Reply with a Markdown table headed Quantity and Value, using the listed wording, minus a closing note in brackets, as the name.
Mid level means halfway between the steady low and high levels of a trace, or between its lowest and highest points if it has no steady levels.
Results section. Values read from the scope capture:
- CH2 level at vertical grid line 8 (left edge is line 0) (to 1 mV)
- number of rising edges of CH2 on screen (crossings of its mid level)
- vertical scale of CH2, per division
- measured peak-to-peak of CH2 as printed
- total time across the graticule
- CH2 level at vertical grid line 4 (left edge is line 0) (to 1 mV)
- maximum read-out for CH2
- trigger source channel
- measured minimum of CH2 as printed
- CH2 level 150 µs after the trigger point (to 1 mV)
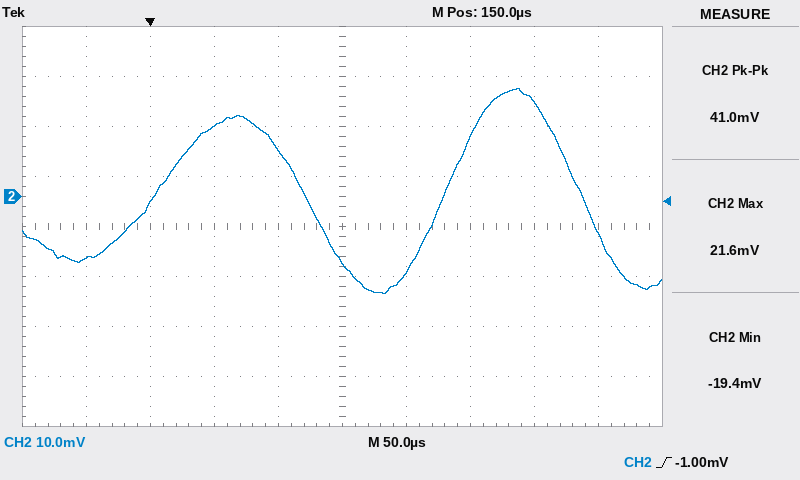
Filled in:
| Quantity | Value |
|---|---|
| CH2 level at vertical grid line 8 (left edge is line 0) | 19 mV |
| number of rising edges of CH2 on screen | 2 |
| vertical scale of CH2, per division | 10 mV |
| measured peak-to-peak of CH2 as printed | 41.0 mV |
| total time across the graticule | 500 µs |
| CH2 level at vertical grid line 4 (left edge is line 0) | 9 mV |
| maximum read-out for CH2 | 21.6 mV |
| trigger source channel | CH2 |
| measured minimum of CH2 as printed | -19.4 mV |
| CH2 level 150 µs after the trigger point | -13 mV |
